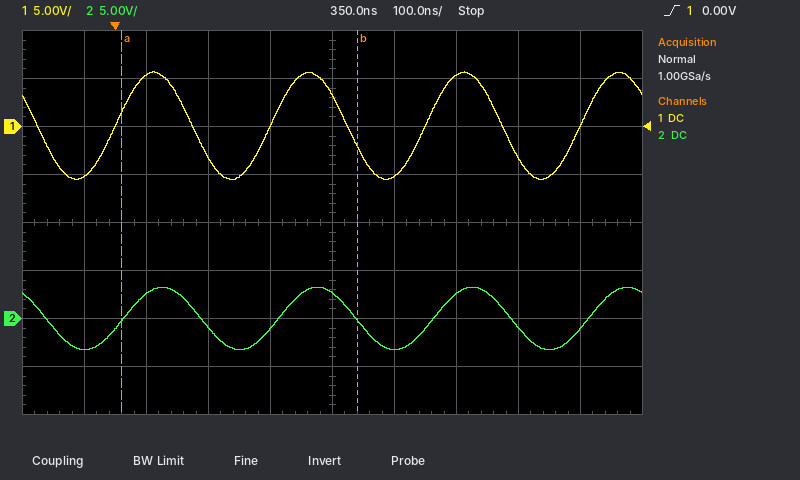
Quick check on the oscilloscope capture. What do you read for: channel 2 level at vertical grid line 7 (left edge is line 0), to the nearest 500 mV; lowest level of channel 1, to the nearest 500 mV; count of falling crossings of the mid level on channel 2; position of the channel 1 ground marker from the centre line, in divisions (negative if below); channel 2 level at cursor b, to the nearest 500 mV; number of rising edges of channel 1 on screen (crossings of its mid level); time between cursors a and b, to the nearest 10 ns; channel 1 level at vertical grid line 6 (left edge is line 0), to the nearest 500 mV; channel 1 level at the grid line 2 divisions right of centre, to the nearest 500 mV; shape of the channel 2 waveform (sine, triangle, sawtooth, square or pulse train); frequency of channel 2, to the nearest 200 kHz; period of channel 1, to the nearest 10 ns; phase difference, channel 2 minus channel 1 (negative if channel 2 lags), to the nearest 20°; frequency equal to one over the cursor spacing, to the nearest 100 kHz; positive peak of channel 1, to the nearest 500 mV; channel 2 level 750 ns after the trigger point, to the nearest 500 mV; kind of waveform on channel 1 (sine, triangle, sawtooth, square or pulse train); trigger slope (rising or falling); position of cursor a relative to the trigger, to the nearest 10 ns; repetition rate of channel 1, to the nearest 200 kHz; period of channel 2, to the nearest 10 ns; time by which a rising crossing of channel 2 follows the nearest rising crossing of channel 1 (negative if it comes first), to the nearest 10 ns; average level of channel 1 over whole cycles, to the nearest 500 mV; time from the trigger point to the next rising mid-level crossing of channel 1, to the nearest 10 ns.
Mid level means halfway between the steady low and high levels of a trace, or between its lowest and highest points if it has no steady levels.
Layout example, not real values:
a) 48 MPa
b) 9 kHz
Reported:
a) 2.5 V
b) -5.5 V
c) 4
d) +2.0 div
e) 0.0 V
f) 4
g) 380 ns
h) -5.0 V
i) 5.5 V
j) sine
k) 4.0 MHz
l) 250 ns
m) -20°
n) 2.6 MHz
o) 5.5 V
p) -1.0 V
q) sine
r) rising
s) +10 ns
t) 4.0 MHz
u) 250 ns
v) +10 ns
w) 0.0 V
x) 250 ns
